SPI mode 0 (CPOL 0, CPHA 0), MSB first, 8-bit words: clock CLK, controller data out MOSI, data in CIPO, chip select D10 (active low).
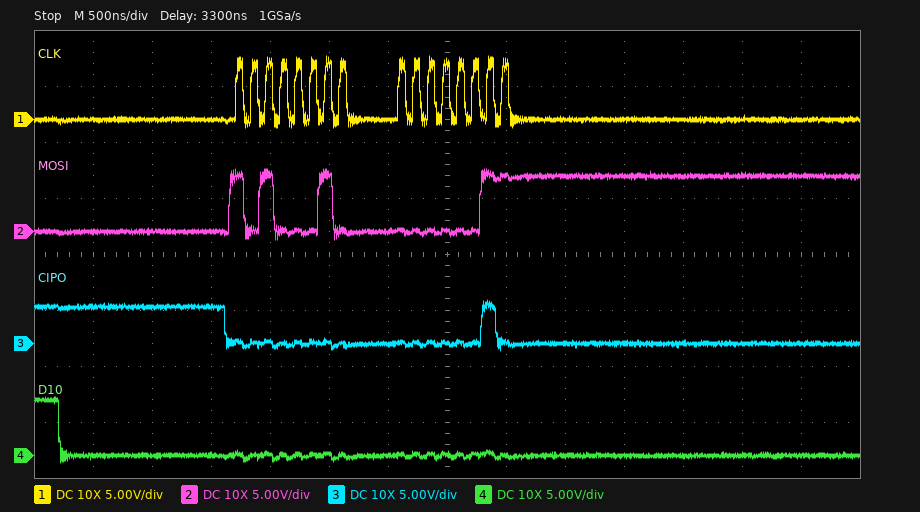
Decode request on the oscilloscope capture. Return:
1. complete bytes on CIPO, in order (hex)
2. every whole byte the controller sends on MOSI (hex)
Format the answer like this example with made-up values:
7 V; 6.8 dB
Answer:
0x00 0x02; 0xA2 0x03
